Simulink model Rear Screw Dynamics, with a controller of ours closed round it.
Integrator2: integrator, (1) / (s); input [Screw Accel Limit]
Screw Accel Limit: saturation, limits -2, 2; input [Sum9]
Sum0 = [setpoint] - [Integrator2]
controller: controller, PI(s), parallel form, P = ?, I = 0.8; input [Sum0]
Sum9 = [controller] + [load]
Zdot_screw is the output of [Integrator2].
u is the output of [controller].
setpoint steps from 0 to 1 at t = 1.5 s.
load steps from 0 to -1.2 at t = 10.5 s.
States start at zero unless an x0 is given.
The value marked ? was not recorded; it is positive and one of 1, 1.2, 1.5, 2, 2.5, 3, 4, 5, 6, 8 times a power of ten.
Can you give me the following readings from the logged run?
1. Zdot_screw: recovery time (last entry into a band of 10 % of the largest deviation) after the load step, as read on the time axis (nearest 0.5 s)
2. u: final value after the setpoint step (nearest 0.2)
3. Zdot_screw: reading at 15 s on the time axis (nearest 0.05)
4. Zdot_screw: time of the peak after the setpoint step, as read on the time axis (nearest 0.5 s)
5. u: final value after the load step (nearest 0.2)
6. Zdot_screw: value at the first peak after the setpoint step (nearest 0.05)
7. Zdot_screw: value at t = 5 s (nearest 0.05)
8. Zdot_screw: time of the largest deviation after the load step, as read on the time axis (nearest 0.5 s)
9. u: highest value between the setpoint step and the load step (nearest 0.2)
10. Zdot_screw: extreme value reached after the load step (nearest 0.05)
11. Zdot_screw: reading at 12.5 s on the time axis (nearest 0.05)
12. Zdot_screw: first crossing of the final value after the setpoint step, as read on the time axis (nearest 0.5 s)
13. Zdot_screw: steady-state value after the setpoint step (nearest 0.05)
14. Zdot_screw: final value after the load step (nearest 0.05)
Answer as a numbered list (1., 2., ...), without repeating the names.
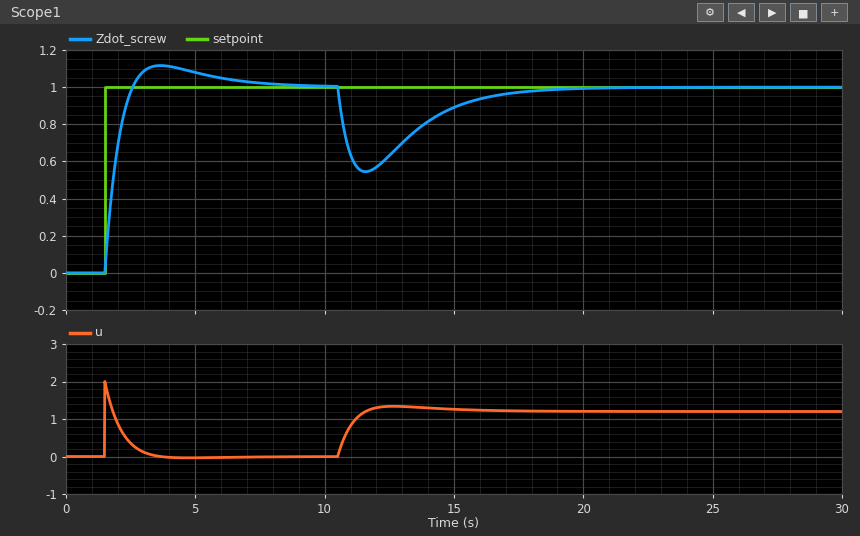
1. 16.5 s
2. 0.0
3. 0.90
4. 3.5 s
5. 1.2
6. 1.10
7. 1.10
8. 11.5 s
9. 2.0
10. 0.55
11. 0.65
12. 2.5 s
13. 1.00
14. 1.00
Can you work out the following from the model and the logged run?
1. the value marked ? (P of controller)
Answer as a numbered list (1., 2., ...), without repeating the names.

1. 2
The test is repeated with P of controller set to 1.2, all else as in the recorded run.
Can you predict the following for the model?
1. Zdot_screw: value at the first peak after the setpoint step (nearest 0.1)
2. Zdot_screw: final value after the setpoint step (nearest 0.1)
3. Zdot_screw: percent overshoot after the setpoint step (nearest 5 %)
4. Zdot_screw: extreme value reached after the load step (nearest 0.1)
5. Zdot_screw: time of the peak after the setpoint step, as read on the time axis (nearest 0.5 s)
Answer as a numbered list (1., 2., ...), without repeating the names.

1. 1.2
2. 1.0
3. 20 %
4. 0.4
5. 4.0 s
